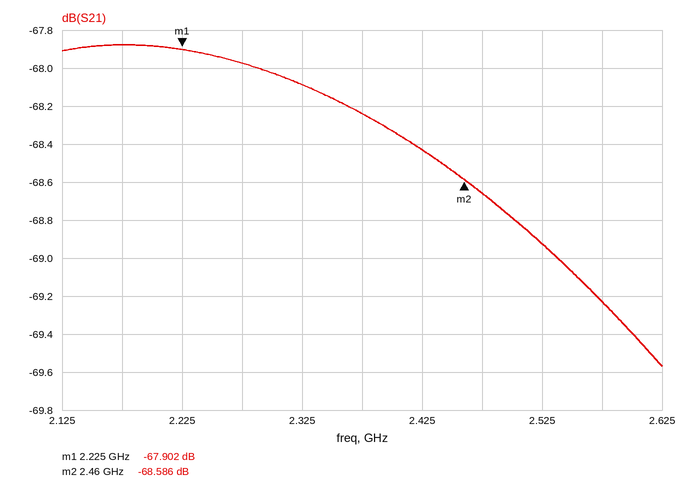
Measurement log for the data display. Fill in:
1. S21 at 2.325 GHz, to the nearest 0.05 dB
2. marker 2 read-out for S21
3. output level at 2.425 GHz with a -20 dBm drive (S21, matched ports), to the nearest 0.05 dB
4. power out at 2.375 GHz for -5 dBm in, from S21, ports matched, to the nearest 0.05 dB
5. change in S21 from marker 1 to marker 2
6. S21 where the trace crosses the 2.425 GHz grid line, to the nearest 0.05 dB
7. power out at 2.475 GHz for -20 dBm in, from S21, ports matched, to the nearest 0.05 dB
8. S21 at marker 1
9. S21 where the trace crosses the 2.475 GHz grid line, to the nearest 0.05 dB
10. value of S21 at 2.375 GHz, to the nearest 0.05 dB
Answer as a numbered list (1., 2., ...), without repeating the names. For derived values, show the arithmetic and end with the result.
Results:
1. -68.10 dB
2. -68.586 dB
3. -20 dBm + (-68.45 dB) = -88.45 dBm
4. -5 dBm + (-68.25 dB) = -73.25 dBm
5. -68.586 − (-67.902) = -0.684 dB
6. -68.45 dB
7. -20 dBm + (-68.65 dB) = -88.65 dBm
8. -67.902 dB
9. -68.65 dB
10. -68.25 dB
